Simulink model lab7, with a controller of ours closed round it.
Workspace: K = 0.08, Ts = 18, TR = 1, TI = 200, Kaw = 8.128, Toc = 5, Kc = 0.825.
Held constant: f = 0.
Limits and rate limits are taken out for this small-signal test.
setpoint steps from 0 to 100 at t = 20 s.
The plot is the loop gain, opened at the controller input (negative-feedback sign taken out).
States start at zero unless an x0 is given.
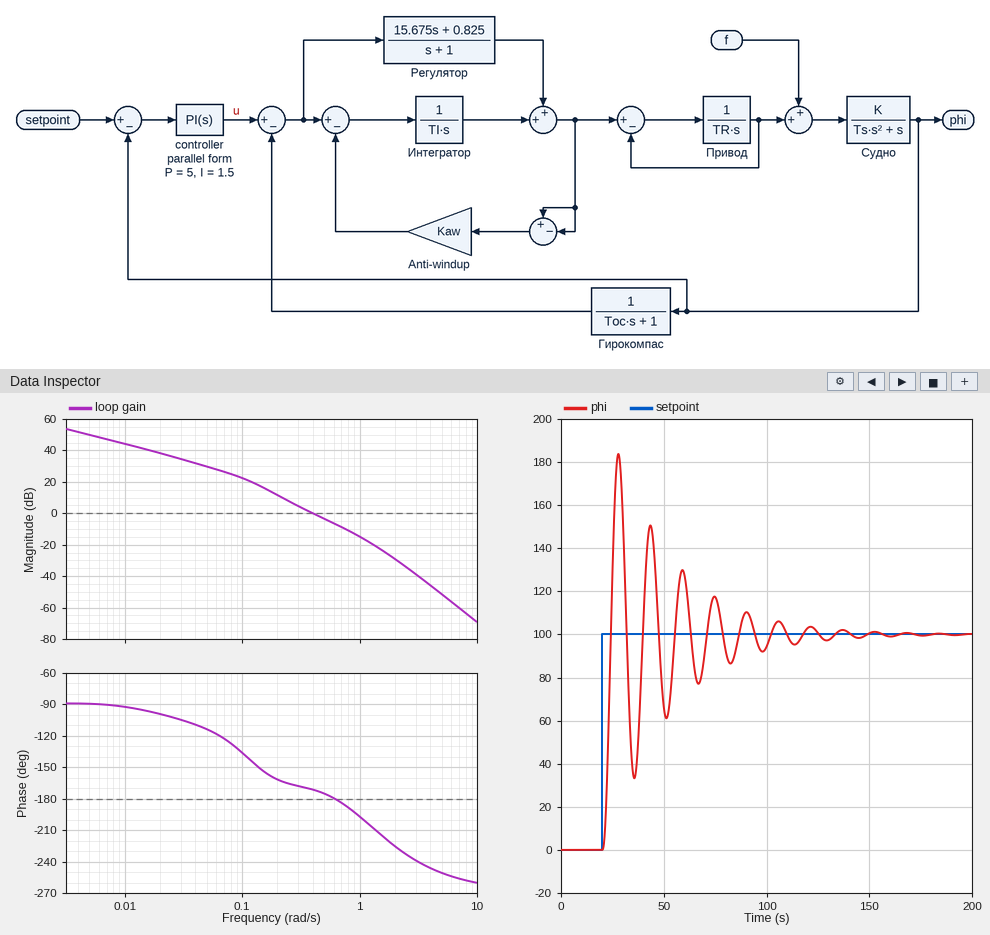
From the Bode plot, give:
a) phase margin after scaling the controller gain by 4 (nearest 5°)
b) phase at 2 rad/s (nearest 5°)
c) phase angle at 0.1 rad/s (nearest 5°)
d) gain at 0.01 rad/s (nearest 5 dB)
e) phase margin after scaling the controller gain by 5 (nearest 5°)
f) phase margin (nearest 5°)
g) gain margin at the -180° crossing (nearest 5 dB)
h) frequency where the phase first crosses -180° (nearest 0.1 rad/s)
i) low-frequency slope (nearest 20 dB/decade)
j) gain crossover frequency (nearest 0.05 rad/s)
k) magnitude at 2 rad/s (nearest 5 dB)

-10°
-225°
-135°
45 dB
-15°
10°
5 dB
0.6 rad/s
-20 dB/decade
0.40 rad/s
-30 dB
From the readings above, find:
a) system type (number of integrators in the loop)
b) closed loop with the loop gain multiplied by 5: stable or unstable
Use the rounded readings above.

1
unstable
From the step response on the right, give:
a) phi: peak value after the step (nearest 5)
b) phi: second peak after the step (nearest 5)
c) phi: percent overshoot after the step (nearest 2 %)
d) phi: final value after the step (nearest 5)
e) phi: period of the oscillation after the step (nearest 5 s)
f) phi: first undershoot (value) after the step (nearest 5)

185
150
84 %
100
15 s
35
